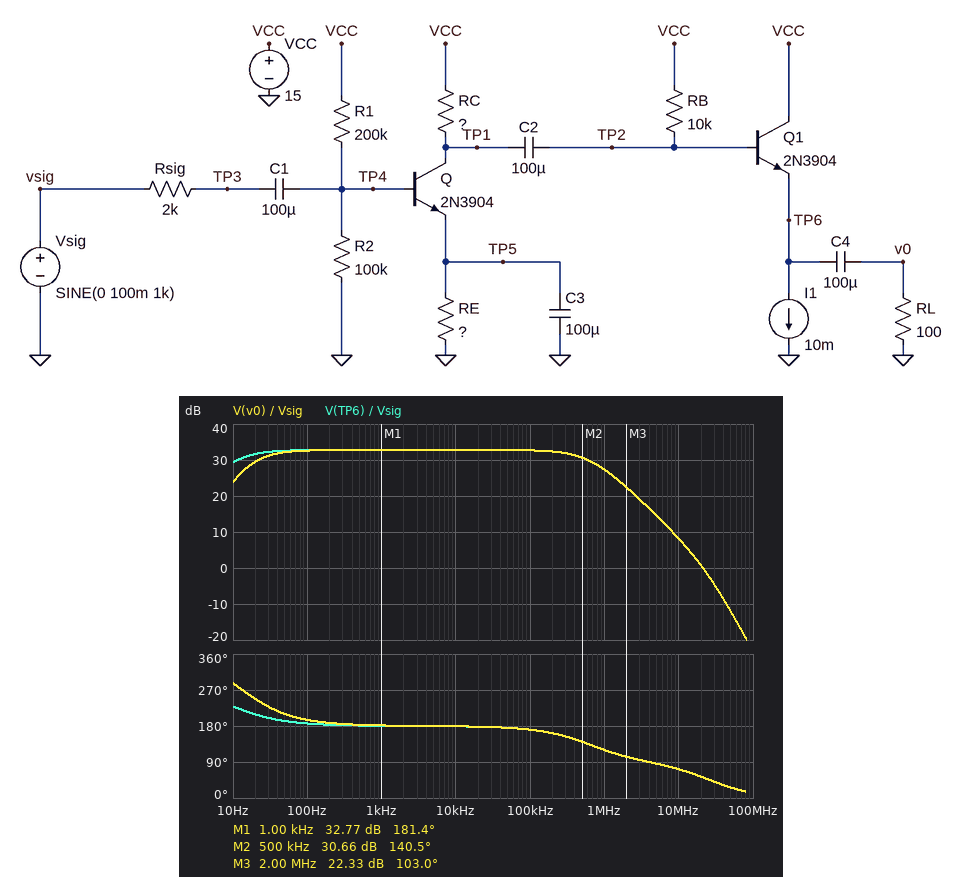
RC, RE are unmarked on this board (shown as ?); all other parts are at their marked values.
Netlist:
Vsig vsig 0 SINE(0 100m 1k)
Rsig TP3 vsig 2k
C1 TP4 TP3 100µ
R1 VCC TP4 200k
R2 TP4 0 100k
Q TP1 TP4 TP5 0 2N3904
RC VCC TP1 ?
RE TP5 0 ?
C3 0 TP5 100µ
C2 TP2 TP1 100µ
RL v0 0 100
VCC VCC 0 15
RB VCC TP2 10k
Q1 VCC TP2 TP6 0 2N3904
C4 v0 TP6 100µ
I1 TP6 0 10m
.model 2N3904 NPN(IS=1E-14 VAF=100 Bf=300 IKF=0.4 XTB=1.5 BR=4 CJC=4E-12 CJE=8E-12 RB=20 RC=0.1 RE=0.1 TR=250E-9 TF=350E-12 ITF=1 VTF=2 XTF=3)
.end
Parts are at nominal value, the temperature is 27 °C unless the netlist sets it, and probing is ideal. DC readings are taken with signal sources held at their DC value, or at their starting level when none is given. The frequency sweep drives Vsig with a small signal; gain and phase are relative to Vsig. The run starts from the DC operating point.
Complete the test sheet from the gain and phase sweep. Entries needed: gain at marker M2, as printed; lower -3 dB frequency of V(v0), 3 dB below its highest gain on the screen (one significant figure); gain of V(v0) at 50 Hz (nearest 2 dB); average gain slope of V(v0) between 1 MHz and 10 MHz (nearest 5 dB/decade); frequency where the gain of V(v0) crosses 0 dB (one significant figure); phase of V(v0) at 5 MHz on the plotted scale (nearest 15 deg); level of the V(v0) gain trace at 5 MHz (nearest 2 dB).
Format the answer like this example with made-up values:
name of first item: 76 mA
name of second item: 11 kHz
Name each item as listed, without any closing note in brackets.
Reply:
gain at marker M2, as printed: 30.66 dB
lower -3 dB frequency of V(v0), 3 dB below its highest gain on the screen: 20 Hz
gain of V(v0) at 50 Hz: 32 dB
average gain slope of V(v0) between 1 MHz and 10 MHz: -20 dB/decade
frequency where the gain of V(v0) crosses 0 dB: 20 MHz
phase of V(v0) at 5 MHz on the plotted scale: 90 deg
level of the V(v0) gain trace at 5 MHz: 14 dB
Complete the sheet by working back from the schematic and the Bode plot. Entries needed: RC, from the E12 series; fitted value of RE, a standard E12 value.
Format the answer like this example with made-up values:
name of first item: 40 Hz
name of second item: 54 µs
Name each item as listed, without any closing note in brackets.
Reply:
RC, from the E12 series: 18 kΩ
fitted value of RE, a standard E12 value: 18 kΩ
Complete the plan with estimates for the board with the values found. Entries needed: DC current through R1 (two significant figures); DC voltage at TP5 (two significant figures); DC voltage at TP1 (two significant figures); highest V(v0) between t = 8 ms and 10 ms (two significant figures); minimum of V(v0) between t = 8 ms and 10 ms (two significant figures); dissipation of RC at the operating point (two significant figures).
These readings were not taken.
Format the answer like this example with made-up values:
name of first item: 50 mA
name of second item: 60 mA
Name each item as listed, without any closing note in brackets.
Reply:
DC current through R1: 50 µA
DC voltage at TP5: 4.3 V
DC voltage at TP1: 11 V
highest V(v0) between t = 8 ms and 10 ms: 930 mV
minimum of V(v0) between t = 8 ms and 10 ms: -1.0 V
dissipation of RC at the operating point: 1.0 mW
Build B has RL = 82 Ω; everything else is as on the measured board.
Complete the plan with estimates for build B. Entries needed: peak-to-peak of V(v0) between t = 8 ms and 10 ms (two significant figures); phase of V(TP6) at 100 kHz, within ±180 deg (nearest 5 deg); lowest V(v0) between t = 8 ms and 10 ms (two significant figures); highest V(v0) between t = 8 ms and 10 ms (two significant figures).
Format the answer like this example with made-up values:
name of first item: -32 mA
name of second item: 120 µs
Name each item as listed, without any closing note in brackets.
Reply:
peak-to-peak of V(v0) between t = 8 ms and 10 ms: 1.7 V
phase of V(TP6) at 100 kHz, within ±180 deg: 170 deg
lowest V(v0) between t = 8 ms and 10 ms: -820 mV
highest V(v0) between t = 8 ms and 10 ms: 870 mV
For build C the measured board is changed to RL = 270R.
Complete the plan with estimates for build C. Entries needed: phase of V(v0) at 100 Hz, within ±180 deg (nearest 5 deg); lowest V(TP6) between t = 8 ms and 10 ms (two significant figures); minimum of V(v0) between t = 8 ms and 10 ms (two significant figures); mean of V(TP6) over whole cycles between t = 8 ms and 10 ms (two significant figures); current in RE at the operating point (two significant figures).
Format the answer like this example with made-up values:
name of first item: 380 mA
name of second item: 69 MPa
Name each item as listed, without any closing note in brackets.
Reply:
phase of V(v0) at 100 Hz, within ±180 deg: -170 deg
lowest V(TP6) between t = 8 ms and 10 ms: 11 V
minimum of V(v0) between t = 8 ms and 10 ms: -2.7 V
mean of V(TP6) over whole cycles between t = 8 ms and 10 ms: 13 V
current in RE at the operating point: 240 µA
